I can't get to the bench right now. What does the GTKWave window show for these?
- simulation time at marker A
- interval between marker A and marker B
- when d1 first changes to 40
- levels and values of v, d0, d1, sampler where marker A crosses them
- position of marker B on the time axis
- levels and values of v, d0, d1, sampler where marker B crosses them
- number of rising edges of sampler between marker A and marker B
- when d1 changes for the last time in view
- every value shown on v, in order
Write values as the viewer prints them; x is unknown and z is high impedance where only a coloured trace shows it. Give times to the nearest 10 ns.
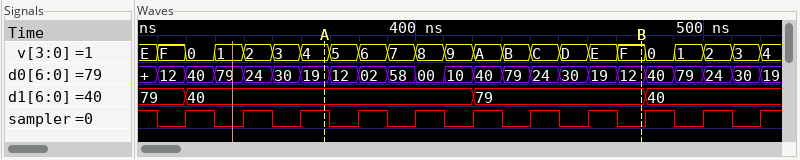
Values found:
370 ns
110 ns
320 ns
v=4, d0=19, d1=40, sampler=1
480 ns
v=F, d0=12, d1=79, sampler=0
5
480 ns
E, F, 0, 1, 2, 3, 4, 5, 6, 7, 8, 9, A, B, C, D, E, F, 0, 1, 2, 3, 4
